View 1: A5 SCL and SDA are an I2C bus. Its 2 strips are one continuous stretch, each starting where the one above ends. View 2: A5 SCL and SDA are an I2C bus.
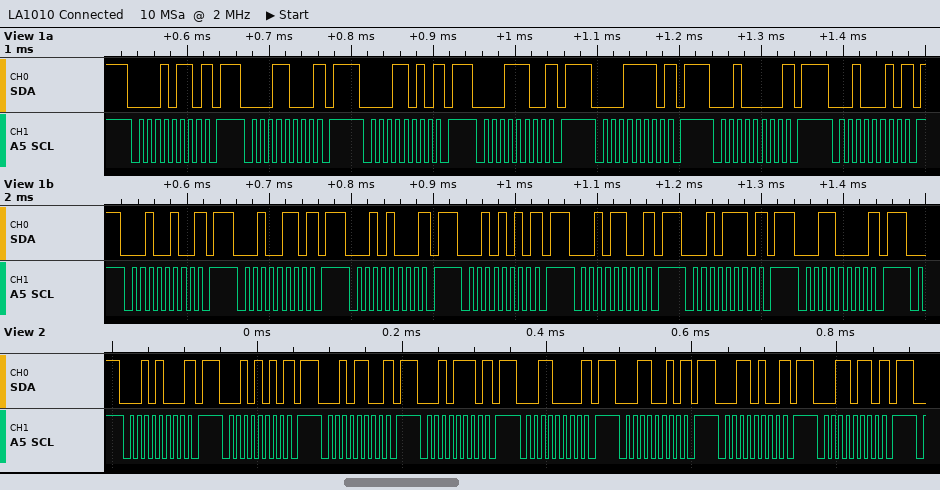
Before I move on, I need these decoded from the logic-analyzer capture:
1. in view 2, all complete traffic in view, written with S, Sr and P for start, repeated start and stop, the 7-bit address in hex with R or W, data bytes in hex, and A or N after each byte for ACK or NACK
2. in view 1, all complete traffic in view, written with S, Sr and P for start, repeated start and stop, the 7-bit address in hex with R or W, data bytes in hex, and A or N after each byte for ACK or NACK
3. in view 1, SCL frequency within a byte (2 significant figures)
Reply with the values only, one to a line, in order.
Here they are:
S 14W N P S 15W N P S 16W N P S 17W N P S 18W N P S 19W N P S 1AW N P S 1BW N P
S 0BW N P S 0CW N P S 0DW N P S 0EW N P S 0FW N P S 10W N P S 11W N P S 12W N P S 13W N P S 14W N P S 15W N P S 16W N P S 17W N P S 18W N P
100 kHz
